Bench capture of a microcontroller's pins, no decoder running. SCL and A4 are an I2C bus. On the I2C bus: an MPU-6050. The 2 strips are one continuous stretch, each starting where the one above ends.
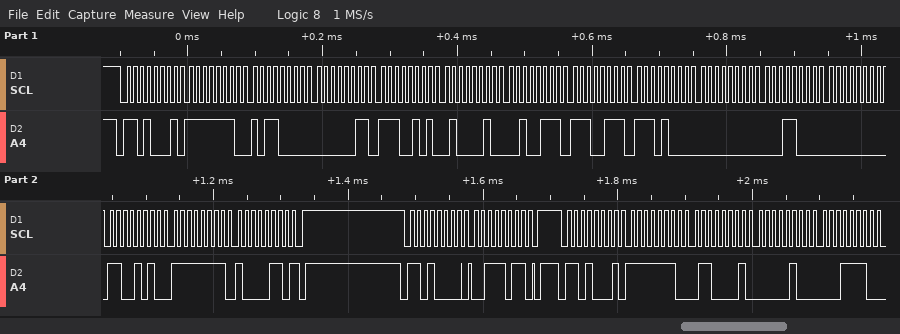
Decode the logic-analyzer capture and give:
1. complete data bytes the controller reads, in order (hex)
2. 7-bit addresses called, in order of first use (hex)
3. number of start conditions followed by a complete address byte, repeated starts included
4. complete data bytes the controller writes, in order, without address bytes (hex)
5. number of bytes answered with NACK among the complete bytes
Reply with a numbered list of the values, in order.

1. FE B0 03 E5 42 27 E7 E8 00 18 00 CA FF 86 FE 61 04 1E
2. 0x68
3. 3
4. 3B
5. 1
